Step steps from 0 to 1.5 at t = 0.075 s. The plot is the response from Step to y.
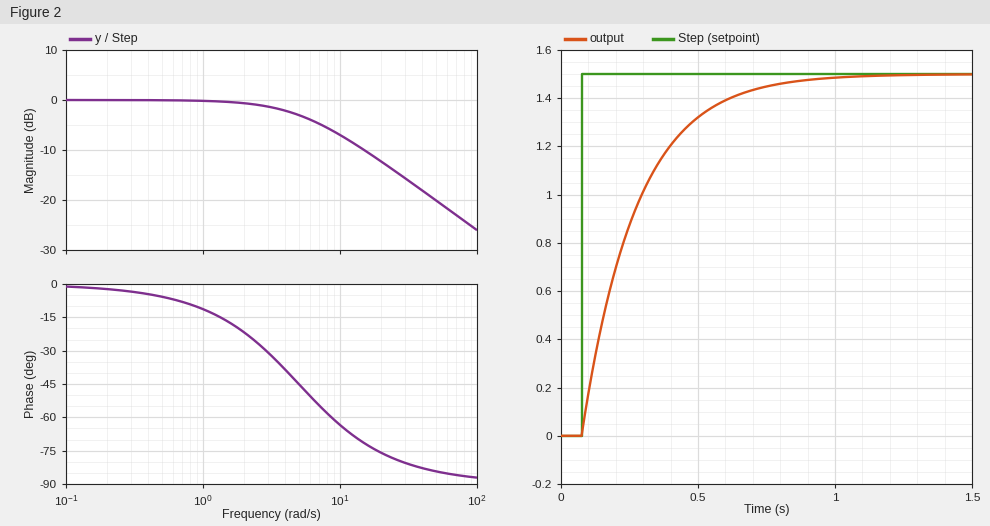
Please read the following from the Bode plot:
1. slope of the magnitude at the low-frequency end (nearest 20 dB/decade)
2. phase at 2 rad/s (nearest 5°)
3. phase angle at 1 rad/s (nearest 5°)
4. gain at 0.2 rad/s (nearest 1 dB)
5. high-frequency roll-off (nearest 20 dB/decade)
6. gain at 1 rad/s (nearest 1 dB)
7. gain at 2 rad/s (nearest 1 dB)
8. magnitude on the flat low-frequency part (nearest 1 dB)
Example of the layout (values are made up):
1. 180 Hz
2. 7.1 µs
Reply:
1. 0 dB/decade
2. -20°
3. -10°
4. 0 dB
5. -20 dB/decade
6. 0 dB
7. -1 dB
8. 0 dB
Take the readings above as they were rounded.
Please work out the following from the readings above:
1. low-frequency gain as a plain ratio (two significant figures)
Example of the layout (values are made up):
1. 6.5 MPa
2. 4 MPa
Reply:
1. 1.0
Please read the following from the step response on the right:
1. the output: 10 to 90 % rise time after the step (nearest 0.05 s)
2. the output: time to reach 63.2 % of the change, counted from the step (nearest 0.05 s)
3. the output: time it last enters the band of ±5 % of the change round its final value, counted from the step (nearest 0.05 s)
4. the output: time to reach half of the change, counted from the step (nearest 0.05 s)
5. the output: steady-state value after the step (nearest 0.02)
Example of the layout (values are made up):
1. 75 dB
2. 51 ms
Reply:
1. 0.45 s
2. 0.20 s
3. 0.60 s
4. 0.15 s
5. 1.50
